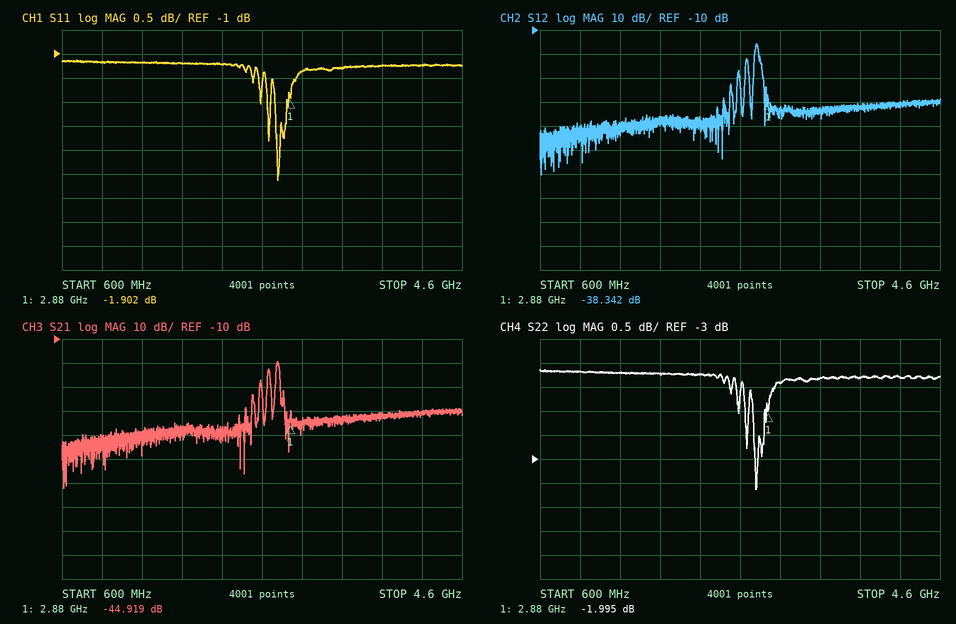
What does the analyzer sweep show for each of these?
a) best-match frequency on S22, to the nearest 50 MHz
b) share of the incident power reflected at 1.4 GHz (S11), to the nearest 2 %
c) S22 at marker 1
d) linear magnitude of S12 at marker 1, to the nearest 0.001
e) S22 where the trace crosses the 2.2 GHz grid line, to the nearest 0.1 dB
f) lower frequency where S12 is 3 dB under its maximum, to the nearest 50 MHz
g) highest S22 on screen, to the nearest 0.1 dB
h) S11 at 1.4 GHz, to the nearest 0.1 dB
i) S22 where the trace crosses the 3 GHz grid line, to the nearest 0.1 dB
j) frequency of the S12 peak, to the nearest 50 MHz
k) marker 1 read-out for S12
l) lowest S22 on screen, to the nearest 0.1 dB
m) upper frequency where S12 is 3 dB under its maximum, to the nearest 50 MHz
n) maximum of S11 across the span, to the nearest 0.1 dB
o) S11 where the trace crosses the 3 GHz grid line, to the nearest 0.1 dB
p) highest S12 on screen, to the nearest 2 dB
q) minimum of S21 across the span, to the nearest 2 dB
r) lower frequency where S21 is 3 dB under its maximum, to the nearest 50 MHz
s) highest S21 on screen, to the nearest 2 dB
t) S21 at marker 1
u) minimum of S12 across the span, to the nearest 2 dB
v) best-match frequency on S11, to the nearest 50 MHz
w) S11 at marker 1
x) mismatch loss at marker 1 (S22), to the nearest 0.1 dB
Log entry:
2.75 GHz
76 %
-1.995 dB
0.012
-1.2 dB
2.75 GHz
-1.1 dB
-1.2 dB
-1.4 dB
2.75 GHz
-38.342 dB
-3.6 dB
2.80 GHz
-1.1 dB
-1.4 dB
-16 dB
-72 dB
2.75 GHz
-20 dB
-44.919 dB
-70 dB
2.75 GHz
-1.902 dB
4.3 dB
